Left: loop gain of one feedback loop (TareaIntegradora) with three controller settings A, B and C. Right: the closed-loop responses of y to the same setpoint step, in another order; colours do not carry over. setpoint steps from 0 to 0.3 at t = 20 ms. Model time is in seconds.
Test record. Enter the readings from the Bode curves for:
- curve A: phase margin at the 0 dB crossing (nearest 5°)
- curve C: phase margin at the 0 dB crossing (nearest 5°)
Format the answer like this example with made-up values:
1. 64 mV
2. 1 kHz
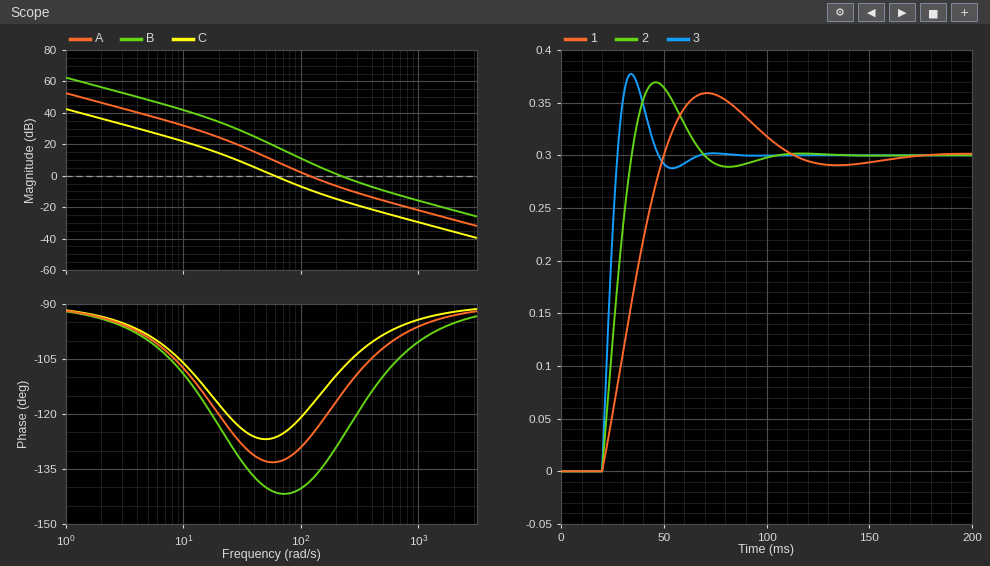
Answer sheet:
1. 55°
2. 55°
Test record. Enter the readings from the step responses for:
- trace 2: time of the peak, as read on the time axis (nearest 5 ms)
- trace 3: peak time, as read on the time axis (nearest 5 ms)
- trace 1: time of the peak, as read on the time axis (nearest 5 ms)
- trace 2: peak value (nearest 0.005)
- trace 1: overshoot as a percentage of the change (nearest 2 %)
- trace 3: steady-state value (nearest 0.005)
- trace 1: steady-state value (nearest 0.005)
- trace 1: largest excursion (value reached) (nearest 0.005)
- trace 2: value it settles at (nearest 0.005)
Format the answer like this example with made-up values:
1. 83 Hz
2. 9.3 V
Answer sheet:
1. 45 ms
2. 35 ms
3. 70 ms
4. 0.370
5. 20 %
6. 0.300
7. 0.300
8. 0.360
9. 0.300
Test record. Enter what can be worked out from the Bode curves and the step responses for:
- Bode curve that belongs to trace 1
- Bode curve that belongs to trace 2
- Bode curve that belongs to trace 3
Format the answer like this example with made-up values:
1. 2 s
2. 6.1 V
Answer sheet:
1. C
2. A
3. B
